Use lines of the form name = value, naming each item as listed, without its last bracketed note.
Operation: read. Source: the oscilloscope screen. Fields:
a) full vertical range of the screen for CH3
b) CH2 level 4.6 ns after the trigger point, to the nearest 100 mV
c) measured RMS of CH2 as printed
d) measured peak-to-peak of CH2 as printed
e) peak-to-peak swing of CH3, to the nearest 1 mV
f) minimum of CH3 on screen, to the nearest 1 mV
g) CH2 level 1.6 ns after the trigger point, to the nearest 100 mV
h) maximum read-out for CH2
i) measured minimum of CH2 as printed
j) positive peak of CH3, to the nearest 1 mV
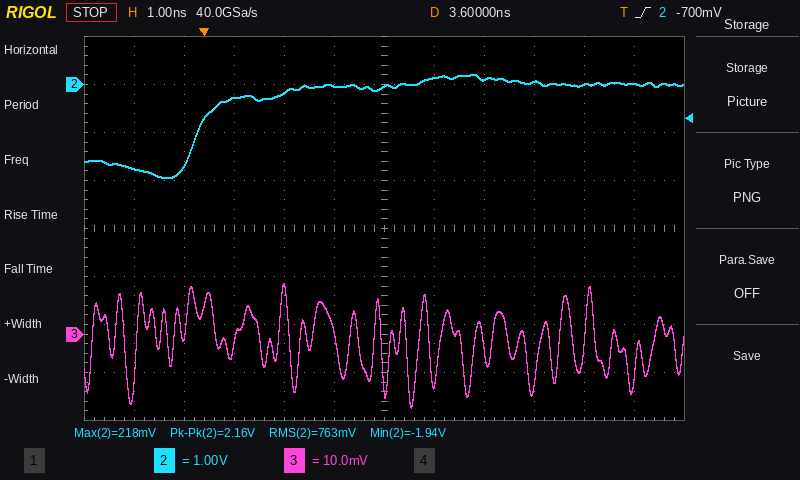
full vertical range of the screen for CH3 = 80 mV
CH2 level 4.6 ns after the trigger point, to the nearest 100 mV = 100 mV
measured RMS of CH2 as printed = 763 mV
measured peak-to-peak of CH2 as printed = 2.16 V
peak-to-peak swing of CH3, to the nearest 1 mV = 26 mV
minimum of CH3 on screen, to the nearest 1 mV = -15 mV
CH2 level 1.6 ns after the trigger point, to the nearest 100 mV = -200 mV
maximum read-out for CH2 = 218 mV
measured minimum of CH2 as printed = -1.94 V
positive peak of CH3, to the nearest 1 mV = 11 mV
